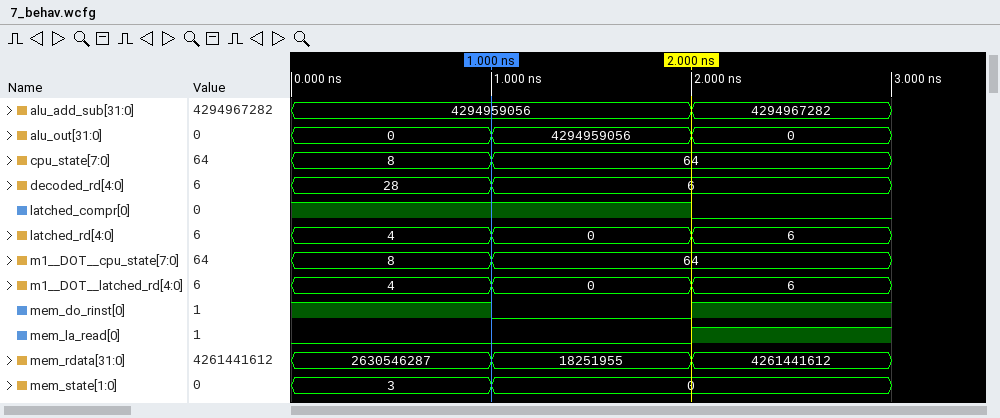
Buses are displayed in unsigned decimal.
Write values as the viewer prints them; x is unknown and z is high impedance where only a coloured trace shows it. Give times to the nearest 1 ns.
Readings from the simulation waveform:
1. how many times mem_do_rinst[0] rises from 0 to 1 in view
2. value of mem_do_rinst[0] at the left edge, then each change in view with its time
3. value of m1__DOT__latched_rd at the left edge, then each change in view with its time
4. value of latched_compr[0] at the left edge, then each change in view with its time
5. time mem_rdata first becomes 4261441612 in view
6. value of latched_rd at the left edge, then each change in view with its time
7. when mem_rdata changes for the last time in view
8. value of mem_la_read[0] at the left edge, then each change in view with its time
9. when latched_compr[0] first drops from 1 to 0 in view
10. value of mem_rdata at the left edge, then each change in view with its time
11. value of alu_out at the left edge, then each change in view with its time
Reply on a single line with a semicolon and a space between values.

1; 1, 0 at 1 ns, 1 at 2 ns; 4, 0 at 1 ns, 6 at 2 ns; 1, 0 at 2 ns; 2 ns; 4, 0 at 1 ns, 6 at 2 ns; 2 ns; 0, 1 at 2 ns; 2 ns; 2630546287, 18251955 at 1 ns, 4261441612 at 2 ns; 0, 4294959056 at 1 ns, 0 at 2 ns
